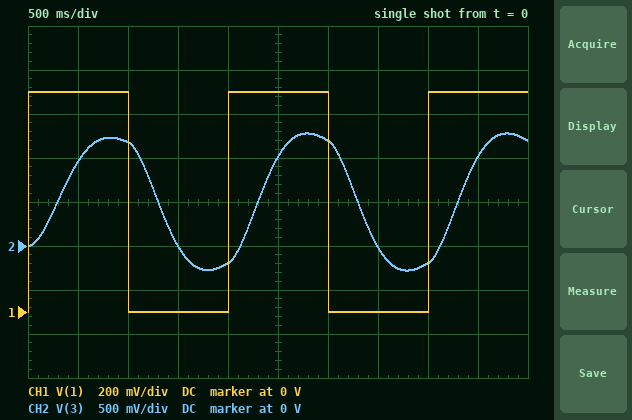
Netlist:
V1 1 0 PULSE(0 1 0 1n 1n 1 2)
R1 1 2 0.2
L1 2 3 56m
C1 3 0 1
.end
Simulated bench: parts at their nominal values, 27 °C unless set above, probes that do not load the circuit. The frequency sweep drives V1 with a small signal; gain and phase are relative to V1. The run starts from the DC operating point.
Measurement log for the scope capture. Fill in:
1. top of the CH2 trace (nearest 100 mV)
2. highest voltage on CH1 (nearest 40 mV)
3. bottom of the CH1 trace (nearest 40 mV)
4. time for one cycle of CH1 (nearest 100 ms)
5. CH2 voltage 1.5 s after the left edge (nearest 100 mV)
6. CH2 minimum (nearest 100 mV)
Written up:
1.3 V
1.00 V
0 V
2.0 s
0 V
-300 mV
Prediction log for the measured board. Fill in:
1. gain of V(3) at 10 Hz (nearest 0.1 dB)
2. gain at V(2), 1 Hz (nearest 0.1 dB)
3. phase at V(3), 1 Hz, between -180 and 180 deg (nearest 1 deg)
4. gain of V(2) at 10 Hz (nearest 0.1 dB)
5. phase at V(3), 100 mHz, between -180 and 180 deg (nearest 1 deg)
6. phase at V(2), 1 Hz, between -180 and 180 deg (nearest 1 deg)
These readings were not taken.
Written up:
-46.9 dB
-3.2 dB
-134 deg
0 dB
-7 deg
46 deg
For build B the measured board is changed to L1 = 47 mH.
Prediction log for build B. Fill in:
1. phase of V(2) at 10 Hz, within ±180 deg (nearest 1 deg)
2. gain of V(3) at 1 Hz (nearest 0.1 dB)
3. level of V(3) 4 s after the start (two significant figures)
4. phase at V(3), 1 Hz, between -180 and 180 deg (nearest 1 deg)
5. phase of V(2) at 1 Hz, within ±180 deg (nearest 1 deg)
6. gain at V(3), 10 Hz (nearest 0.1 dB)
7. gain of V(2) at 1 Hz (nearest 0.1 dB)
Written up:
4 deg
-3.6 dB
-120 mV
-124 deg
56 deg
-45.3 dB
-5.0 dB
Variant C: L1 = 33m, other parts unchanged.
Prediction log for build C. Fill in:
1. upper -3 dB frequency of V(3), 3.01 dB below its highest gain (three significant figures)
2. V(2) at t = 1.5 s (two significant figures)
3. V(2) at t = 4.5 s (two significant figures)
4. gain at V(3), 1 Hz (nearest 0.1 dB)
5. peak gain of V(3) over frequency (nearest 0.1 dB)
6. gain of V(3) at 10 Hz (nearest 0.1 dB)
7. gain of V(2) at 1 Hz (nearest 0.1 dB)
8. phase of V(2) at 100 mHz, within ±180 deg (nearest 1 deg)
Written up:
1.00 Hz
210 mV
790 mV
-2.2 dB
0.7 dB
-42.3 dB
-12.6 dB
-7 deg
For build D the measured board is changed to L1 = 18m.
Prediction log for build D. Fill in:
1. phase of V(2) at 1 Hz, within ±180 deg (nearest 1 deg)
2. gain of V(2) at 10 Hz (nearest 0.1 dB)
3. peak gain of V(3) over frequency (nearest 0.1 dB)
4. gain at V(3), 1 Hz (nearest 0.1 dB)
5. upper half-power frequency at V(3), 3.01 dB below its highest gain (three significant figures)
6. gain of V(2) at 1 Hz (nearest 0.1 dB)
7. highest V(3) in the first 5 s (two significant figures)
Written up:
-77 deg
-0.1 dB
0 dB
-2.2 dB
1.12 Hz
-13.0 dB
1.0 V
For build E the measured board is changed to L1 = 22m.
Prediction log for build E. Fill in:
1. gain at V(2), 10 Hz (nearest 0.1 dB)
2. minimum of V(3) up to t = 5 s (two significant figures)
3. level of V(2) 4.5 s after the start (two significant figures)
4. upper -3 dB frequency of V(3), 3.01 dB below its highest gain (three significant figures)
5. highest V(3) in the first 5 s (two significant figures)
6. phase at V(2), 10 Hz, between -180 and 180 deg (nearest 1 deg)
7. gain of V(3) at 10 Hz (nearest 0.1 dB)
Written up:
-0.1 dB
-57 mV
890 mV
1.12 Hz
1.1 V
8 deg
-38.8 dB
